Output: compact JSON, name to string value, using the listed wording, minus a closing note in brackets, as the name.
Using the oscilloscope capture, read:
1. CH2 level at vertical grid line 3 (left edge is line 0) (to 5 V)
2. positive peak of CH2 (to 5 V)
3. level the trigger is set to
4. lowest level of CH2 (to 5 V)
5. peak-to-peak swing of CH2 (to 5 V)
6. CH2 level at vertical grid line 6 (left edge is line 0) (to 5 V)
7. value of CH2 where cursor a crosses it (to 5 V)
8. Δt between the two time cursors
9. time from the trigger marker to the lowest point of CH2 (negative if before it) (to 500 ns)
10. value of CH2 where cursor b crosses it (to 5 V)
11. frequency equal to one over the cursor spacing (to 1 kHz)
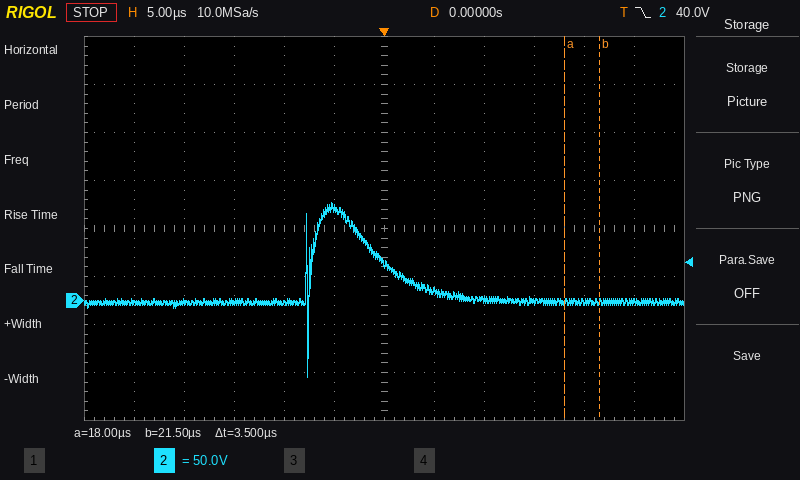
{"CH2 level at vertical grid line 3 (left edge is line 0)": "0 V", "positive peak of CH2": "100 V", "level the trigger is set to": "40.0 V", "lowest level of CH2": "-80 V", "peak-to-peak swing of CH2": "180 V", "CH2 level at vertical grid line 6 (left edge is line 0)": "40 V", "value of CH2 where cursor a crosses it": "0 V", "Δt between the two time cursors": "3.5 µs", "time from the trigger marker to the lowest point of CH2 (negative if before it)": "-7.5 µs", "value of CH2 where cursor b crosses it": "0 V", "frequency equal to one over the cursor spacing": "286 kHz"}
